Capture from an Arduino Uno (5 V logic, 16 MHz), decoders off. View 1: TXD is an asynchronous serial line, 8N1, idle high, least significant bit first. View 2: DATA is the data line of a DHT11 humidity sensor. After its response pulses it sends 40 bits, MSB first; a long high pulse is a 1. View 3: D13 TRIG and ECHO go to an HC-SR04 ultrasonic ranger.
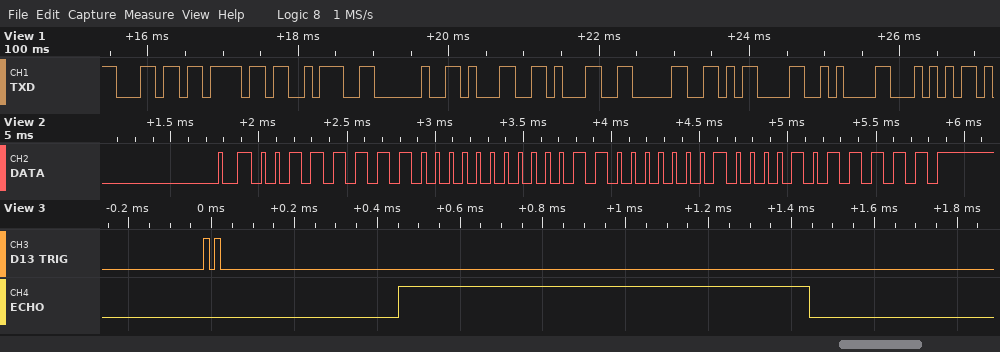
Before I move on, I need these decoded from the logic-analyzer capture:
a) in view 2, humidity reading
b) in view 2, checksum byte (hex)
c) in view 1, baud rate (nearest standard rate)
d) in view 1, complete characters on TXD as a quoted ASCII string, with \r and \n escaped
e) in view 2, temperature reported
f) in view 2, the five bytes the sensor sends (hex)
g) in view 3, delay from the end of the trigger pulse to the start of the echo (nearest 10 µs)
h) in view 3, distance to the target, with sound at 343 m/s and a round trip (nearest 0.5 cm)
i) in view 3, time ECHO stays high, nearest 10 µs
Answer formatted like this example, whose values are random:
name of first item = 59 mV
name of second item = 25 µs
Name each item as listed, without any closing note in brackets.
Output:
in view 2, humidity reading = 63 %
in view 2, checksum byte = 0x5F
in view 1, baud rate = 9600 baud
in view 1, complete characters on TXD as a quoted ASCII string, with \r and \n escaped = "lo: 110\r\nT"
in view 2, temperature reported = 24.8 °C
in view 2, the five bytes the sensor sends = 3F 00 18 08 5F
in view 3, delay from the end of the trigger pulse to the start of the echo = 430 µs
in view 3, distance to the target, with sound at 343 m/s and a round trip = 17 cm
in view 3, time ECHO stays high, nearest 10 µs = 990 µs
